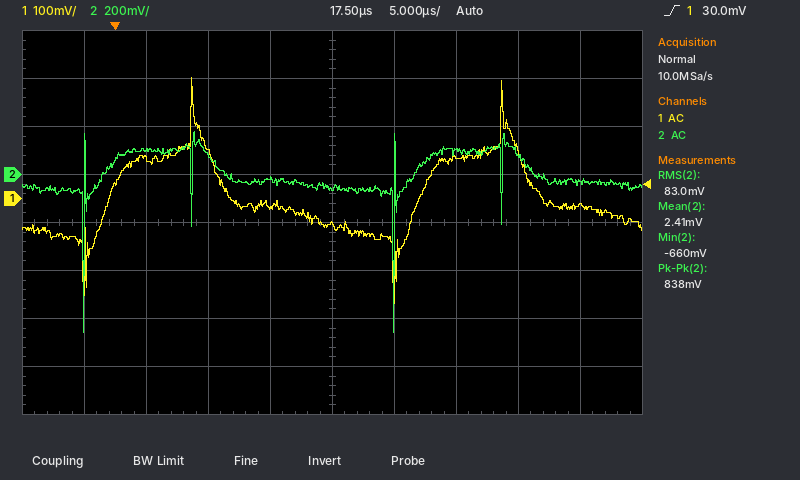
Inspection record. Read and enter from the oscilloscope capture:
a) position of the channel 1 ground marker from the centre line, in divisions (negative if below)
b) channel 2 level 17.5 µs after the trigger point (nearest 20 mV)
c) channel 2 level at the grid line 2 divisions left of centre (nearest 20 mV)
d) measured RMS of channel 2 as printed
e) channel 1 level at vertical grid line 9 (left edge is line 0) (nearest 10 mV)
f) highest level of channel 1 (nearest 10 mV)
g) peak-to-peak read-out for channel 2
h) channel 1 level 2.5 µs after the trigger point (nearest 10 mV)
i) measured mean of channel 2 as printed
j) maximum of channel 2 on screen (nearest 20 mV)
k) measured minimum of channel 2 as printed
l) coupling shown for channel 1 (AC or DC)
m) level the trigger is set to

+0.5 div
-60 mV
80 mV
83.0 mV
-10 mV
250 mV
838 mV
80 mV
2.41 mV
180 mV
-660 mV
AC
30.0 mV
